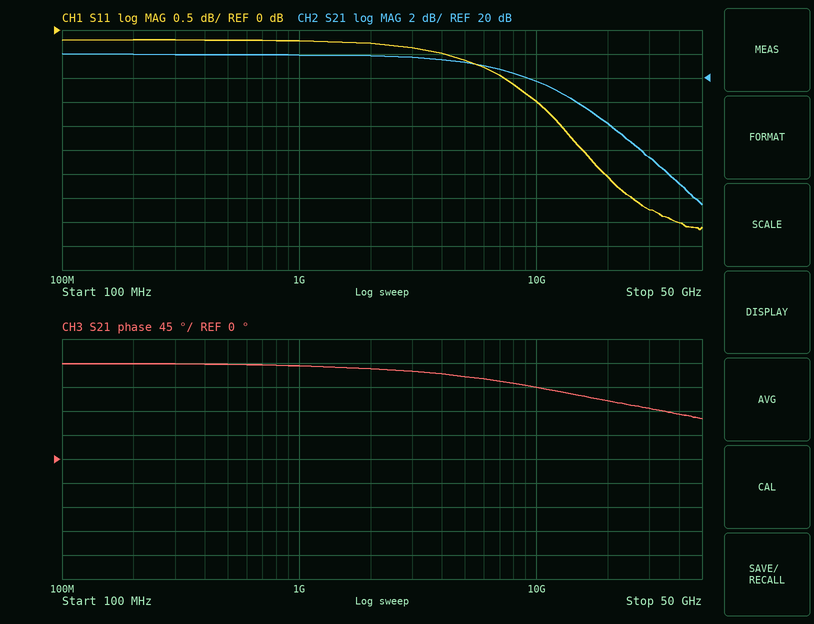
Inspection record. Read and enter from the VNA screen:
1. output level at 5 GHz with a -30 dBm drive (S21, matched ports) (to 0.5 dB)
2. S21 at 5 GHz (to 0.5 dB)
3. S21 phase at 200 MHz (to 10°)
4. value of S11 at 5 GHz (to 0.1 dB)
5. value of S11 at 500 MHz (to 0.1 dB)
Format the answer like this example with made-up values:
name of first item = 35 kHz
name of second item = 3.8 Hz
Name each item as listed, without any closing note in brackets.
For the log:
output level at 5 GHz with a -30 dBm drive (S21, matched ports) = -8.5 dBm
S21 at 5 GHz = 21.5 dB
S21 phase at 200 MHz = 180°
value of S11 at 5 GHz = -0.6 dB
value of S11 at 500 MHz = -0.2 dB
